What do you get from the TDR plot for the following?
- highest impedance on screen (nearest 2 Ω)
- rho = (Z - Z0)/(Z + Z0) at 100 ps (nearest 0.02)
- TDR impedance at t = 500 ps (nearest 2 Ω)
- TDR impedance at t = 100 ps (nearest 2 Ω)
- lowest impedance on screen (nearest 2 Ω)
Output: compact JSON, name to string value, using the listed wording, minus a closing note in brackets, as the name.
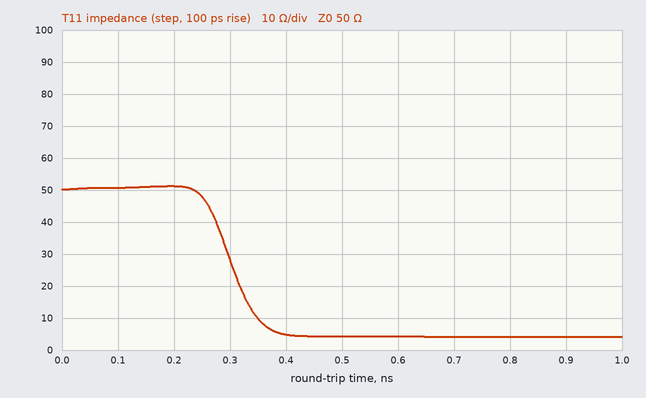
{"highest impedance on screen": "52 Ω", "rho = (Z - Z0)/(Z + Z0) at 100 ps": "0.00", "TDR impedance at t = 500 ps": "4 Ω", "TDR impedance at t = 100 ps": "50 Ω", "lowest impedance on screen": "4 Ω"}
